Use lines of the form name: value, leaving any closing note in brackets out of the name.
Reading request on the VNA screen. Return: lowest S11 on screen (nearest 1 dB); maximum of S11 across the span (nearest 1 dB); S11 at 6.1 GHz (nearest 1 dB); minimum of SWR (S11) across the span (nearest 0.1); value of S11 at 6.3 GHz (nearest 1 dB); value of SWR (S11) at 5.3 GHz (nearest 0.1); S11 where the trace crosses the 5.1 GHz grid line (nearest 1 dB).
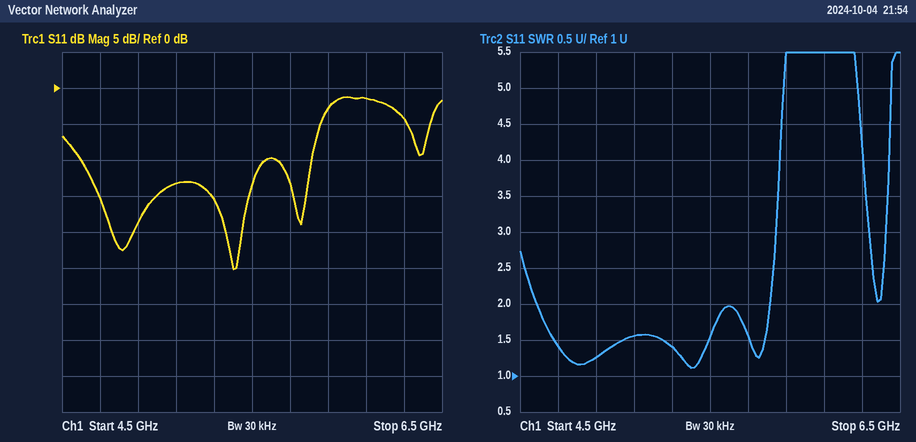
lowest S11 on screen: -25 dB
maximum of S11 across the span: -1 dB
S11 at 6.1 GHz: -1 dB
minimum of SWR (S11) across the span: 1.1
value of S11 at 6.3 GHz: -4 dB
value of SWR (S11) at 5.3 GHz: 1.4
S11 where the trace crosses the 5.1 GHz grid line: -13 dB
